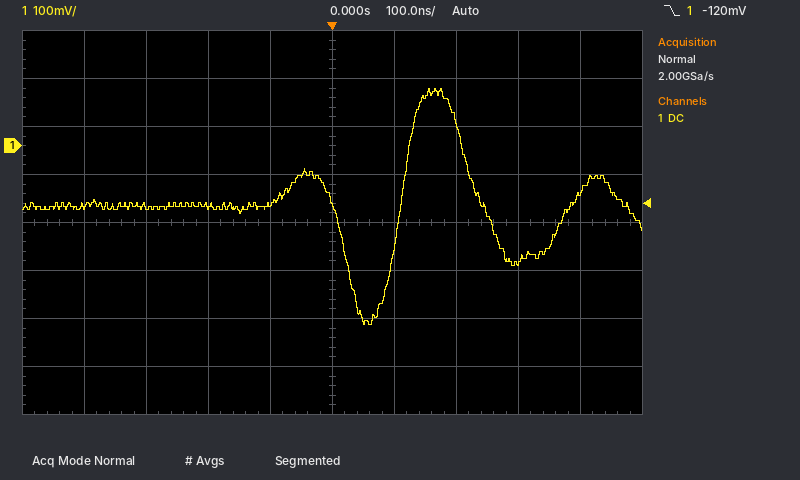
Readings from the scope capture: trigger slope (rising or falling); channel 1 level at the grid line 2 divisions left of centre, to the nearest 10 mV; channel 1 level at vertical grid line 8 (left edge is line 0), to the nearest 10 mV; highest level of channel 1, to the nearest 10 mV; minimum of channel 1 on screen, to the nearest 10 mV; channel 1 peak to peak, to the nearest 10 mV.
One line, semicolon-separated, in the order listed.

falling; -130 mV; -240 mV; 120 mV; -370 mV; 490 mV
